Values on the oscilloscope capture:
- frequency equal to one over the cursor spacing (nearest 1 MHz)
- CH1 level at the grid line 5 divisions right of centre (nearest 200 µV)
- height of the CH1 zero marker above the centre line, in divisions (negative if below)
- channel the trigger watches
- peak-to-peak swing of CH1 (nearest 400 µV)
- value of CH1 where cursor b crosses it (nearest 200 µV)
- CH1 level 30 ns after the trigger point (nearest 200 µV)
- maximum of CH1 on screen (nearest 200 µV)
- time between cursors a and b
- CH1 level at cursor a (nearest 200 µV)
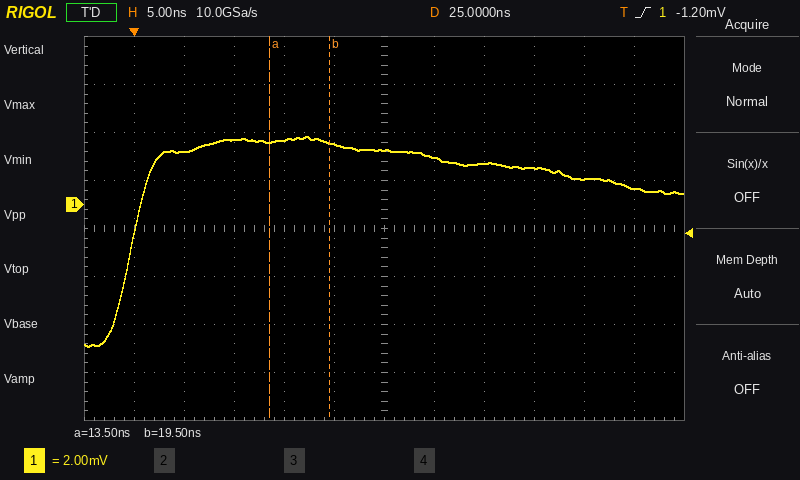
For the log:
167 MHz
600 µV
+0.5 div
CH1
8.8 mV
2.6 mV
2.0 mV
2.8 mV
6.0 ns
2.6 mV
